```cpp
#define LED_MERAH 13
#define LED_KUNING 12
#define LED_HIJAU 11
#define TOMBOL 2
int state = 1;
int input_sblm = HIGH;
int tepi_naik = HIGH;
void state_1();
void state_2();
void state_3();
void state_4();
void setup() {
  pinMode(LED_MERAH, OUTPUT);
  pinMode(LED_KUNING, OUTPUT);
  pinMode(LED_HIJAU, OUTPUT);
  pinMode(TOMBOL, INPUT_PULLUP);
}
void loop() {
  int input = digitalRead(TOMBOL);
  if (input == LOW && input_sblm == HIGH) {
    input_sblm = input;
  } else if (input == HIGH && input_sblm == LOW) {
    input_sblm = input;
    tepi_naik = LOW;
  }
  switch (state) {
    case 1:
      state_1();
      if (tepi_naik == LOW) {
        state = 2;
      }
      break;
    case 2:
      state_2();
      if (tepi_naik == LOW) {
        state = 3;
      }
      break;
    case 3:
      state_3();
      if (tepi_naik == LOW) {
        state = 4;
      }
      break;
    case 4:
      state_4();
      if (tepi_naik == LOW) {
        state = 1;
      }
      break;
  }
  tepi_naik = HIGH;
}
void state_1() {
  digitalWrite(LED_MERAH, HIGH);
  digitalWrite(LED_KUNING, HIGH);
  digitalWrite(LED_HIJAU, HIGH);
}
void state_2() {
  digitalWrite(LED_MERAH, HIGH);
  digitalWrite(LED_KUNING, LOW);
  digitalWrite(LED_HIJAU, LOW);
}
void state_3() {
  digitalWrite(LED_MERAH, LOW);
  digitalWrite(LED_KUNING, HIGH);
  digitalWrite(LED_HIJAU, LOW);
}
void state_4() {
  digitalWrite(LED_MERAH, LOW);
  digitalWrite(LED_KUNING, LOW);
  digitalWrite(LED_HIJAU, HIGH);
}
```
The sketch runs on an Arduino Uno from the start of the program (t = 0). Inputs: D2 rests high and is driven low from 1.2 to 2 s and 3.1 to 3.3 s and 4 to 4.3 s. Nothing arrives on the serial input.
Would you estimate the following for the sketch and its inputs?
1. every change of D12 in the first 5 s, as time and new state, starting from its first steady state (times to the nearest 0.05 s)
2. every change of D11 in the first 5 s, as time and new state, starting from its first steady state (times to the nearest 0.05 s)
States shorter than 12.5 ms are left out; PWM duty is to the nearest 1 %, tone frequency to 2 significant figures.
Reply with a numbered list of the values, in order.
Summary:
1. 0 s high; 2 s low; 3.3 s high; 4.3 s low
2. 0 s high; 2 s low; 4.3 s high
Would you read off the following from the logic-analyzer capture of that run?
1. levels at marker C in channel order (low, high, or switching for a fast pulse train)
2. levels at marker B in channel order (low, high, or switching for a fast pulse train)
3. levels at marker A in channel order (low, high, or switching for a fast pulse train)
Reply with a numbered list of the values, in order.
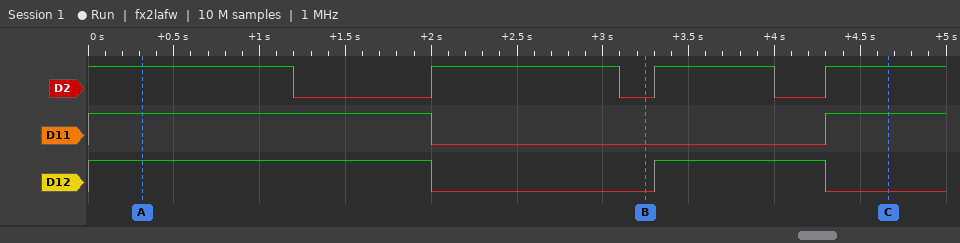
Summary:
1. D2 high, D11 high, D12 low
2. D2 low, D11 low, D12 low
3. D2 high, D11 high, D12 high
